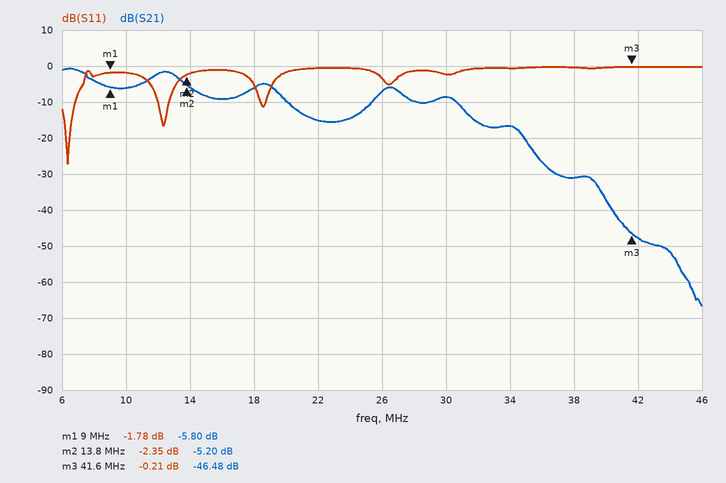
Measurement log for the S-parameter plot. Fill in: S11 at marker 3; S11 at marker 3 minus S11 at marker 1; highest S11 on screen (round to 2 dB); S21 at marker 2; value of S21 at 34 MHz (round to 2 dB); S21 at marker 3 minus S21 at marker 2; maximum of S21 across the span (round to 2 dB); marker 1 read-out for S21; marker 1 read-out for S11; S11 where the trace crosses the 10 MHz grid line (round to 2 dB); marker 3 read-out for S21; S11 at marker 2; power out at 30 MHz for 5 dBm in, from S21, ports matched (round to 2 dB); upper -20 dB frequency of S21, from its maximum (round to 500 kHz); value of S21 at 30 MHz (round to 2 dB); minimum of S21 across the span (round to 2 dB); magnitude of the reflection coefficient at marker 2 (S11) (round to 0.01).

-0.21 dB
1.57 dB
0 dB
-5.20 dB
-16 dB
-41.28 dB
0 dB
-5.80 dB
-1.78 dB
-2 dB
-46.48 dB
-2.35 dB
-4 dBm
35.0 MHz
-8 dB
-66 dB
0.76
